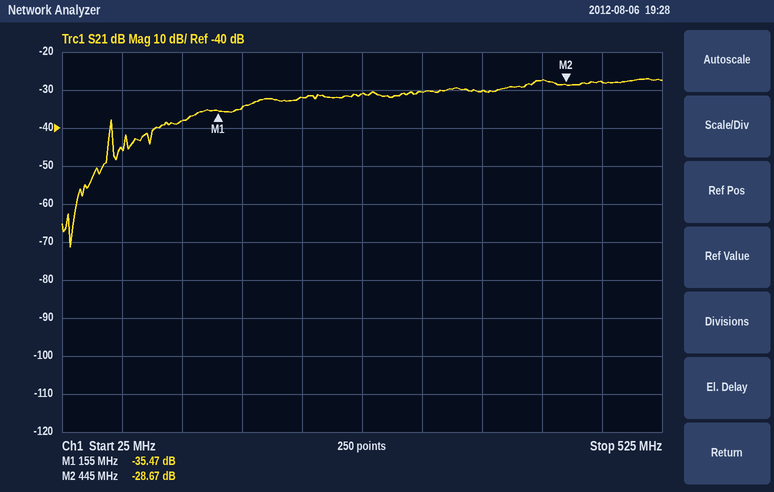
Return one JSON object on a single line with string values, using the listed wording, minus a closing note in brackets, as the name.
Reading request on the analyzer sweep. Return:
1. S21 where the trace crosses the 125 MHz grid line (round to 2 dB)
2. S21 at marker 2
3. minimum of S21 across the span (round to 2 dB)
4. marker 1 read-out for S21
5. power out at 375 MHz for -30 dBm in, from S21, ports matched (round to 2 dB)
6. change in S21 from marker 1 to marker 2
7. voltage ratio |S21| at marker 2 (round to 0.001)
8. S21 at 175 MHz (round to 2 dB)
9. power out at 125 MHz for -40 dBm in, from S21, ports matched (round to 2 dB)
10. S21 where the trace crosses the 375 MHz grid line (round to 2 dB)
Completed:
{"S21 where the trace crosses the 125 MHz grid line": "-38 dB", "S21 at marker 2": "-28.67 dB", "minimum of S21 across the span": "-72 dB", "marker 1 read-out for S21": "-35.47 dB", "power out at 375 MHz for -30 dBm in, from S21, ports matched": "-60 dBm", "change in S21 from marker 1 to marker 2": "6.80 dB", "voltage ratio |S21| at marker 2": "0.037", "S21 at 175 MHz": "-34 dB", "power out at 125 MHz for -40 dBm in, from S21, ports matched": "-78 dBm", "S21 where the trace crosses the 375 MHz grid line": "-30 dB"}
